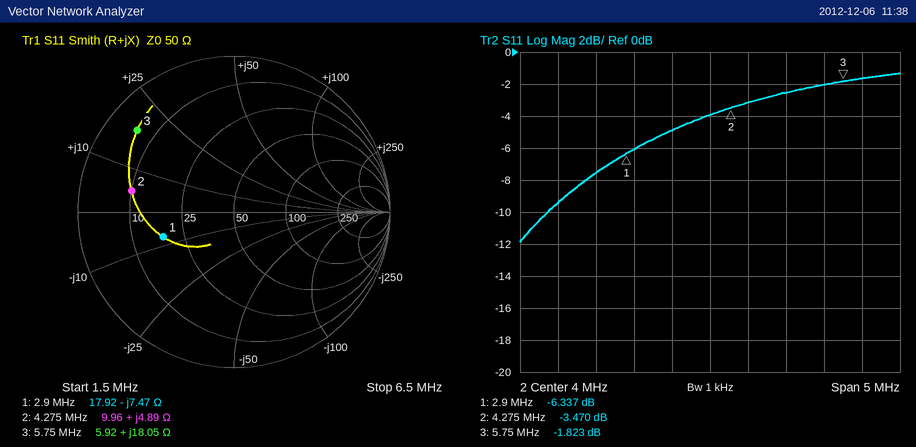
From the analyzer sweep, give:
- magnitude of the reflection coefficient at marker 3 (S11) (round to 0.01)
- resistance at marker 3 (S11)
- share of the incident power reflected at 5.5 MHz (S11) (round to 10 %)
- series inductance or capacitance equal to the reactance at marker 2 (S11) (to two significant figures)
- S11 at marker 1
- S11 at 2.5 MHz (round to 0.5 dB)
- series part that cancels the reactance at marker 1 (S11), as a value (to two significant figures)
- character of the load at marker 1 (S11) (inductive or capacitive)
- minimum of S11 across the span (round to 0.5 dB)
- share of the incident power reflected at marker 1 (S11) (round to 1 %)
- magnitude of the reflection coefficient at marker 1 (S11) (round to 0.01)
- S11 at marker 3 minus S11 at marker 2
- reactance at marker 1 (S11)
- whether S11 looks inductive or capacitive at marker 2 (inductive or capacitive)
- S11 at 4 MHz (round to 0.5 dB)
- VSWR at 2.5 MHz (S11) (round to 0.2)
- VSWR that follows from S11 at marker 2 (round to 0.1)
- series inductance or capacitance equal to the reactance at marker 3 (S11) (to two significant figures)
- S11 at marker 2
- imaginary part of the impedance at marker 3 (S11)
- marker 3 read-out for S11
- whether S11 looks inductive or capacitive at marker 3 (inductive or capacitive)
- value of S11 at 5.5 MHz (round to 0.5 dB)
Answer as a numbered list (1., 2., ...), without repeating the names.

1. 0.81
2. 5.92 Ω
3. 60 %
4. 180 nH
5. -6.337 dB
6. -7.5 dB
7. 410 nH
8. capacitive
9. -12.0 dB
10. 23 %
11. 0.48
12. 1.647 dB
13. -7.47 Ω
14. inductive
15. -4.0 dB
16. 2.4
17. 5.1
18. 500 nH
19. -3.470 dB
20. +18.05 Ω
21. -1.823 dB
22. inductive
23. -2.0 dB
